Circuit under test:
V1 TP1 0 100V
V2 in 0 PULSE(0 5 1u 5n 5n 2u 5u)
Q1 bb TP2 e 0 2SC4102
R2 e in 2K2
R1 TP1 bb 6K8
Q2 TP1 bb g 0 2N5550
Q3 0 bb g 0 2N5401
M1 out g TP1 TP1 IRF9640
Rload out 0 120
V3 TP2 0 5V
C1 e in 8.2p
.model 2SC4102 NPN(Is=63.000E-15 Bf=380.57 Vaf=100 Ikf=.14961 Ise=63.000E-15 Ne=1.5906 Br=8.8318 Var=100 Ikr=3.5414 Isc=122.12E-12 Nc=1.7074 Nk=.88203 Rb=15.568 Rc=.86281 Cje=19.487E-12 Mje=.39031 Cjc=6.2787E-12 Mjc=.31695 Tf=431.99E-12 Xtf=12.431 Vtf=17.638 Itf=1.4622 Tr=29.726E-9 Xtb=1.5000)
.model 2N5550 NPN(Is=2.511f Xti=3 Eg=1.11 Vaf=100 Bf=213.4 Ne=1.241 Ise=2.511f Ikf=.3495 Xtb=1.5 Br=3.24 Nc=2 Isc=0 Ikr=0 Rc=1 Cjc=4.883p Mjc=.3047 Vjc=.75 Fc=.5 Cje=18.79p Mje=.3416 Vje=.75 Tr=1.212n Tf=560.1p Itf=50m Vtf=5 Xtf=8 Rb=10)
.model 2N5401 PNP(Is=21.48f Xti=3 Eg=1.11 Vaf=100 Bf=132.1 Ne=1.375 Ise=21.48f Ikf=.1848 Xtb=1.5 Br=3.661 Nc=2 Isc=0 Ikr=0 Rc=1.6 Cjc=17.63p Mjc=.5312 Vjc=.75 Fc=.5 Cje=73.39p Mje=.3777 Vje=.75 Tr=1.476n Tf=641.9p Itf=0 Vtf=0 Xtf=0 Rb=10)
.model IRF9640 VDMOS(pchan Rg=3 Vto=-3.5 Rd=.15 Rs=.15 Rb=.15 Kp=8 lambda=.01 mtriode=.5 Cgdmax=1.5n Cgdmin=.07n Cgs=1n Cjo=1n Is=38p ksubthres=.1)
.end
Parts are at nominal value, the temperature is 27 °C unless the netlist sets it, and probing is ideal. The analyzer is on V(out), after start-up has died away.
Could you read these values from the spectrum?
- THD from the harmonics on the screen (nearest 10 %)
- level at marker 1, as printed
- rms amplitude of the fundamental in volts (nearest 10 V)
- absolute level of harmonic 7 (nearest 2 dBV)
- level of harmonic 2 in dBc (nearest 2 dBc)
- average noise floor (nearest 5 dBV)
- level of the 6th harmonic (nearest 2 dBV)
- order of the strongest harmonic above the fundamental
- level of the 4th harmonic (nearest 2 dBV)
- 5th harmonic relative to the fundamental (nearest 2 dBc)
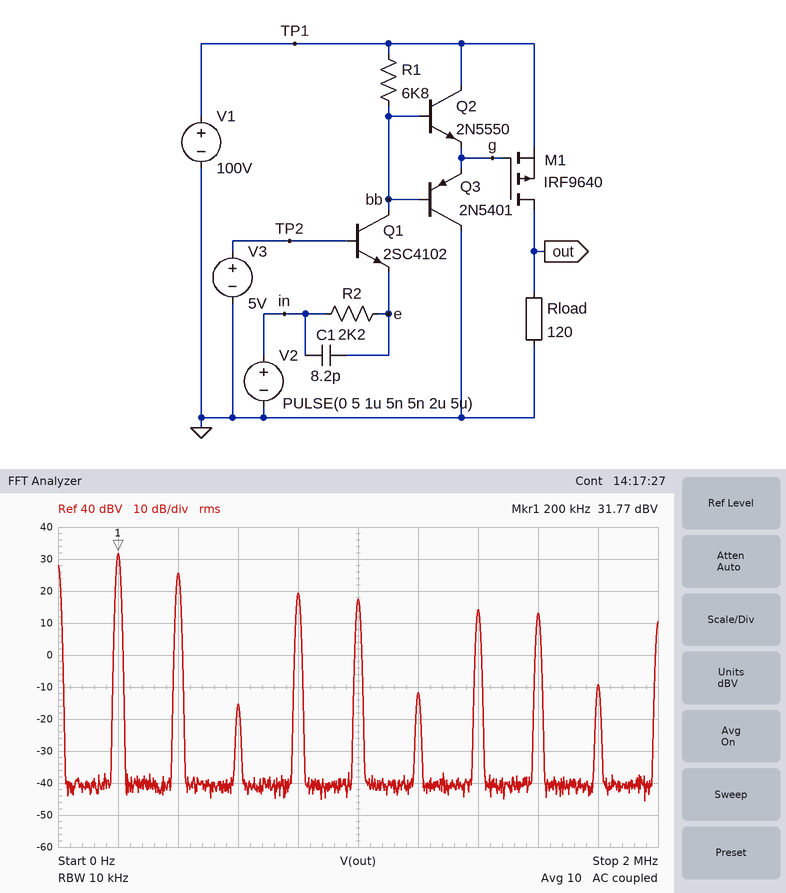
60 %
31.77 dBV
40 V
14 dBV
-6 dBc
-40 dBV
-12 dBV
2
20 dBV
-14 dBc
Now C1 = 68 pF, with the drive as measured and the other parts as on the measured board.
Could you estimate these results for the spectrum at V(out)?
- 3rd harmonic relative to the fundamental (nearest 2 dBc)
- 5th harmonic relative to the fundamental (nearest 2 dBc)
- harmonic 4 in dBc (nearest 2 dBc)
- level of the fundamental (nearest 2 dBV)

-22 dBc
-12 dBc
-14 dBc
32 dBV
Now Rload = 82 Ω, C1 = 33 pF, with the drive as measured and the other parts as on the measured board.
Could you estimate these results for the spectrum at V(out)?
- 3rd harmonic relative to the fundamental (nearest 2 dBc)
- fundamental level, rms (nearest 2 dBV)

-28 dBc
32 dBV
